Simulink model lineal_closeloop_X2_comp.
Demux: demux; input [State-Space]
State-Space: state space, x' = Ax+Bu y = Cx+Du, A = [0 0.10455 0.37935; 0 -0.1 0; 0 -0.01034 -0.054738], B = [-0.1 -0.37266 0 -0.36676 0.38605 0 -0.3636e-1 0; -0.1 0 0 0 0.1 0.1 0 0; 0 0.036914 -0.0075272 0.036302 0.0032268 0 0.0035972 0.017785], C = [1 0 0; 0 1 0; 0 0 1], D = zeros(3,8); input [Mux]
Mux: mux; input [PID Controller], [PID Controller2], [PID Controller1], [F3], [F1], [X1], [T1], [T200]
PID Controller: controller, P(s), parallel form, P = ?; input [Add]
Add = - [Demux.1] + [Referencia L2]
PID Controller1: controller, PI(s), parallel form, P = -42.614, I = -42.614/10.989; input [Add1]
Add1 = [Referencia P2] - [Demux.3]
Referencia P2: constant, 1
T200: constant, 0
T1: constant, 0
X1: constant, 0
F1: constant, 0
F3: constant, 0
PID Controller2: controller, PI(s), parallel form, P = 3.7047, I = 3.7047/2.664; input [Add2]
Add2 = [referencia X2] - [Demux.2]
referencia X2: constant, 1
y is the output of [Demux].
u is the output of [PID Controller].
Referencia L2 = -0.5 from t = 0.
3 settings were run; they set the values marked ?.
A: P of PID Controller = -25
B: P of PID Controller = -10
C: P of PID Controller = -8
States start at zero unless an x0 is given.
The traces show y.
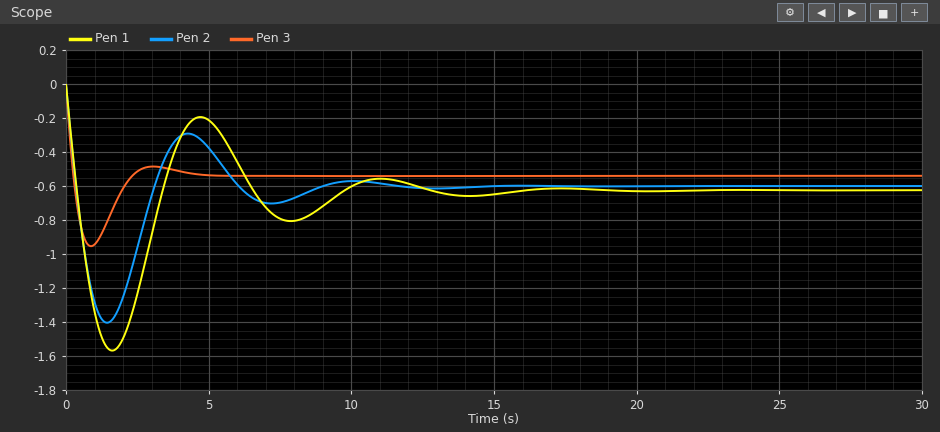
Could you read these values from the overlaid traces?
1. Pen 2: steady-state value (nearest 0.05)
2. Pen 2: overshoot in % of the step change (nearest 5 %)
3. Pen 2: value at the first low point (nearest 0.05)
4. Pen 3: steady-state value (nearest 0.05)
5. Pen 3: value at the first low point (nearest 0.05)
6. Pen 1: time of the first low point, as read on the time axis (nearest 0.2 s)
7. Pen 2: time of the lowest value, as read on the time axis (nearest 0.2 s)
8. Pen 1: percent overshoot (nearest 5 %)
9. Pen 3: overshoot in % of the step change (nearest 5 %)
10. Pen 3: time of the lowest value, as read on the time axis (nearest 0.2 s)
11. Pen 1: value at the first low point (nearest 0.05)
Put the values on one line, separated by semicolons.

-0.60; 135 %; -1.40; -0.55; -0.95; 1.6 s; 1.4 s; 150 %; 75 %; 0.8 s; -1.55
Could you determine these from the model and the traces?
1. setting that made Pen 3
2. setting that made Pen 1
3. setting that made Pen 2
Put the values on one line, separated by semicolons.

A; C; B
